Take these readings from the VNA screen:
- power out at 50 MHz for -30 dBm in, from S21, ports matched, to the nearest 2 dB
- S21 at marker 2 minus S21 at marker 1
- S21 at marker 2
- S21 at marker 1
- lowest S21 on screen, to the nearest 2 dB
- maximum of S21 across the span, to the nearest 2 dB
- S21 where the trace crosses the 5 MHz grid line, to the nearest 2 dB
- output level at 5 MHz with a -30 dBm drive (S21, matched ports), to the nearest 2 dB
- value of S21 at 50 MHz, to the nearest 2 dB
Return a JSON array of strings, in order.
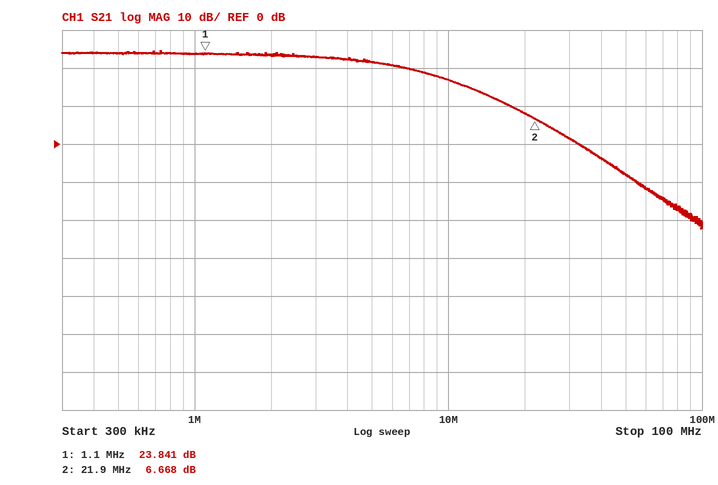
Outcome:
["-38 dBm", "-17.173 dB", "6.668 dB", "23.841 dB", "-22 dB", "24 dB", "22 dB", "-8 dBm", "-8 dB"]
